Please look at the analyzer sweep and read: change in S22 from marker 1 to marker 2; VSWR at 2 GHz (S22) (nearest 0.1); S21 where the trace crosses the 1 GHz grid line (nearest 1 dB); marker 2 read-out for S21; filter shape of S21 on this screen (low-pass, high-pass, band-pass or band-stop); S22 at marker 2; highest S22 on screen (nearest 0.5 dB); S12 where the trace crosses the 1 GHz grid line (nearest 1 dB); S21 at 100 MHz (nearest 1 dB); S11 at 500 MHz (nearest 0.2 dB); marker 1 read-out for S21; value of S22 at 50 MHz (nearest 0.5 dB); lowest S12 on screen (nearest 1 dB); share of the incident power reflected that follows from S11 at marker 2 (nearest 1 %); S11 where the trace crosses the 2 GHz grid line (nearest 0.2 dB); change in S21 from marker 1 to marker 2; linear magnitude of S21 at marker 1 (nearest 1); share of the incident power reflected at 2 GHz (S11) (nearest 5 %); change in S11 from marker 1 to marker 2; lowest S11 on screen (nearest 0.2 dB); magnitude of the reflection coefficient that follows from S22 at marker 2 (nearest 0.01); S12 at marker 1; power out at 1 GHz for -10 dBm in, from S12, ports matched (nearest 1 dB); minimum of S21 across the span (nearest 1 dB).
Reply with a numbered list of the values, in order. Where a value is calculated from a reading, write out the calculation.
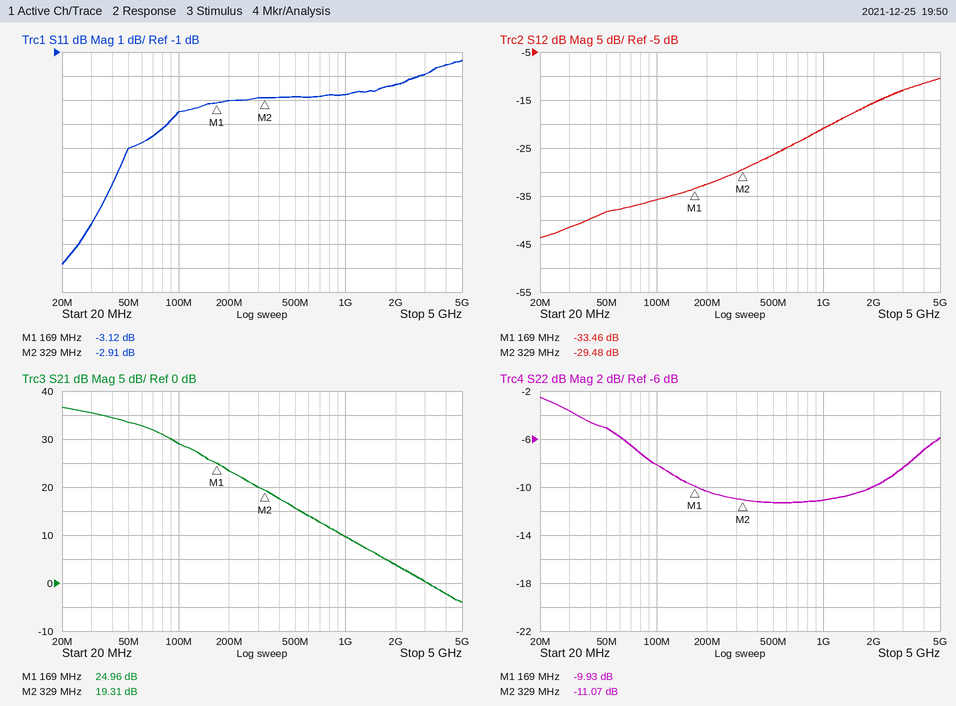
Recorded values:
1. -11.07 − (-9.93) = -1.14 dB
2. |Γ| = 10^(-10/20) = 0.3162; VSWR = (1 + 0.3162)/(1 − 0.3162) ≈ 1.9
3. 10 dB
4. 19.31 dB
5. low-pass
6. -11.07 dB
7. -2.5 dB
8. -21 dB
9. 29 dB
10. -2.8 dB
11. 24.96 dB
12. -5.0 dB
13. -44 dB
14. 10^(-2.91/10) ≈ 51 %
15. -2.4 dB
16. 19.31 − (24.96) = -5.65 dB
17. 10^(24.96/20) ≈ 18
18. 10^(-2.4/10) ≈ 57.5 %, so 60 % to the nearest 5 %
19. -2.91 − (-3.12) = 0.21 dB
20. -9.8 dB
21. 10^(-11.07/20) ≈ 0.28
22. -33.46 dB
23. -10 dBm + (-21 dB) = -31 dBm
24. -4 dB
